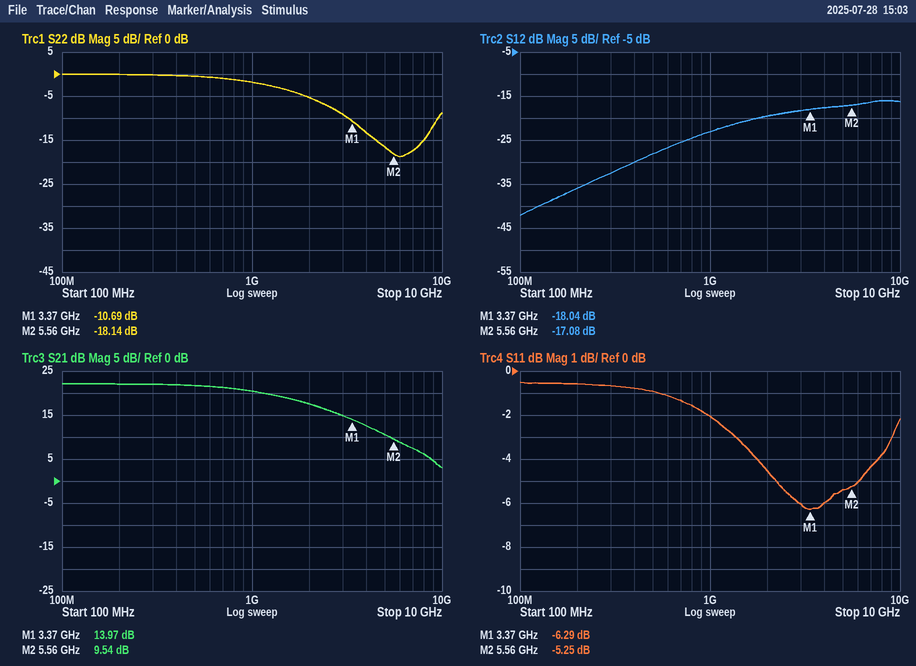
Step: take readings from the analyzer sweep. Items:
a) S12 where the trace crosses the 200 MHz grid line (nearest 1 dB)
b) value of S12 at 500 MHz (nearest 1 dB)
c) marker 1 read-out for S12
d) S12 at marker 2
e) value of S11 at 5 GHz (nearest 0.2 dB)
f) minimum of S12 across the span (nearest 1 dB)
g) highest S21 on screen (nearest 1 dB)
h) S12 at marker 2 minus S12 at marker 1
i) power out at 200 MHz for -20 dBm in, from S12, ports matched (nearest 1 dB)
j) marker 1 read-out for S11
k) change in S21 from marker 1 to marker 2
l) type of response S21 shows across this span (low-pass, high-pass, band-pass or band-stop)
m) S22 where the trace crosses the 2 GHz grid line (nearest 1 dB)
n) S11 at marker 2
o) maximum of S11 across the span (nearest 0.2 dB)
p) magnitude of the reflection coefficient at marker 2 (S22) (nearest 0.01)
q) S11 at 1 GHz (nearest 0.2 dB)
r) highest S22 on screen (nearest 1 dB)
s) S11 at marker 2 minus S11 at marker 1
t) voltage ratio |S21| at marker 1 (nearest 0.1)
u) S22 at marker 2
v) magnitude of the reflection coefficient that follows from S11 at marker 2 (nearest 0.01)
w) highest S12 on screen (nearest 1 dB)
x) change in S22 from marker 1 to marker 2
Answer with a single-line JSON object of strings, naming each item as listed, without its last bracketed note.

{"S12 where the trace crosses the 200 MHz grid line": "-36 dB", "value of S12 at 500 MHz": "-28 dB", "marker 1 read-out for S12": "-18.04 dB", "S12 at marker 2": "-17.08 dB", "value of S11 at 5 GHz": "-5.4 dB", "minimum of S12 across the span": "-42 dB", "highest S21 on screen": "22 dB", "S12 at marker 2 minus S12 at marker 1": "0.96 dB", "power out at 200 MHz for -20 dBm in, from S12, ports matched": "-56 dBm", "marker 1 read-out for S11": "-6.29 dB", "change in S21 from marker 1 to marker 2": "-4.43 dB", "type of response S21 shows across this span": "low-pass", "S22 where the trace crosses the 2 GHz grid line": "-5 dB", "S11 at marker 2": "-5.25 dB", "maximum of S11 across the span": "-0.6 dB", "magnitude of the reflection coefficient at marker 2 (S22)": "0.12", "S11 at 1 GHz": "-2.0 dB", "highest S22 on screen": "0 dB", "S11 at marker 2 minus S11 at marker 1": "1.04 dB", "voltage ratio |S21| at marker 1": "5.0", "S22 at marker 2": "-18.14 dB", "magnitude of the reflection coefficient that follows from S11 at marker 2": "0.55", "highest S12 on screen": "-16 dB", "change in S22 from marker 1 to marker 2": "-7.45 dB"}
